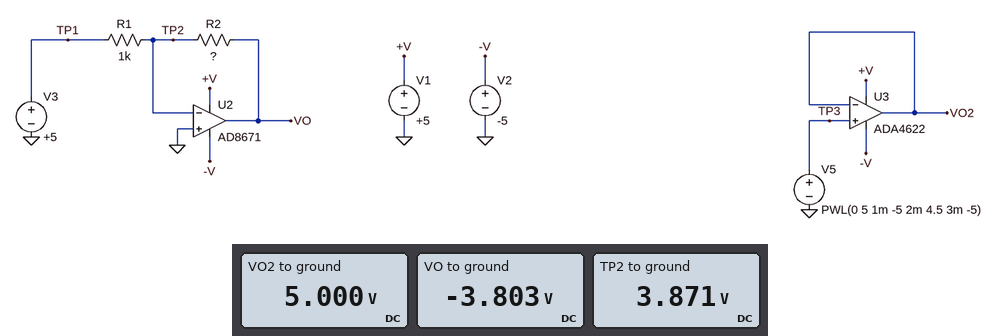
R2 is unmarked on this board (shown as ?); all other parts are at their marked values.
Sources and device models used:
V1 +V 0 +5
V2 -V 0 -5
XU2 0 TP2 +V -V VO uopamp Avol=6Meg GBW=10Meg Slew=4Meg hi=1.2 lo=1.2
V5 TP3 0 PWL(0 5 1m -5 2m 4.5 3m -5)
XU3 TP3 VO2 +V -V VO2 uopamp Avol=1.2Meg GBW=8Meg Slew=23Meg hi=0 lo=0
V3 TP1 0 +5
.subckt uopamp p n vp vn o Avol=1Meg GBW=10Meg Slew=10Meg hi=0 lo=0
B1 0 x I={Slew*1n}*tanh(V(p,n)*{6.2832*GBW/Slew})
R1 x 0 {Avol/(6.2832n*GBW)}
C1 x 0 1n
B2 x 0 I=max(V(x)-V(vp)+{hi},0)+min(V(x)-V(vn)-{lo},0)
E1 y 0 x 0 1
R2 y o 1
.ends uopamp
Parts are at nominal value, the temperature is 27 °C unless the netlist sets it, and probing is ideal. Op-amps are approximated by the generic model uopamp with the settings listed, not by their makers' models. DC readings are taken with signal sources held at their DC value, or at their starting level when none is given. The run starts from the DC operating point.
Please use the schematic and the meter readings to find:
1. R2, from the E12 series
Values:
6.8 kΩ
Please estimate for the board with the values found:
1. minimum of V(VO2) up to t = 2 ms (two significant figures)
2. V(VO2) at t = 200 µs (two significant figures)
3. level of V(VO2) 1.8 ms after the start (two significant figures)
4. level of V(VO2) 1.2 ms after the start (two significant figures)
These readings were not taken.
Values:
-5.0 V
3.0 V
2.6 V
-3.1 V
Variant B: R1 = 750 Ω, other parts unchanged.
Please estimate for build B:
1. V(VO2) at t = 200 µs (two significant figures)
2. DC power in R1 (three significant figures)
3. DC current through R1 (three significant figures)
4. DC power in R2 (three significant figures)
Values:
3.0 V
1.02 mW
1.17 mA
9.24 mW
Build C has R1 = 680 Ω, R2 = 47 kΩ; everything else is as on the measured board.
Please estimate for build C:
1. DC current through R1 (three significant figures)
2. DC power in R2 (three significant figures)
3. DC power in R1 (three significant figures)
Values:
185 µA
1.60 mW
23.2 µW
